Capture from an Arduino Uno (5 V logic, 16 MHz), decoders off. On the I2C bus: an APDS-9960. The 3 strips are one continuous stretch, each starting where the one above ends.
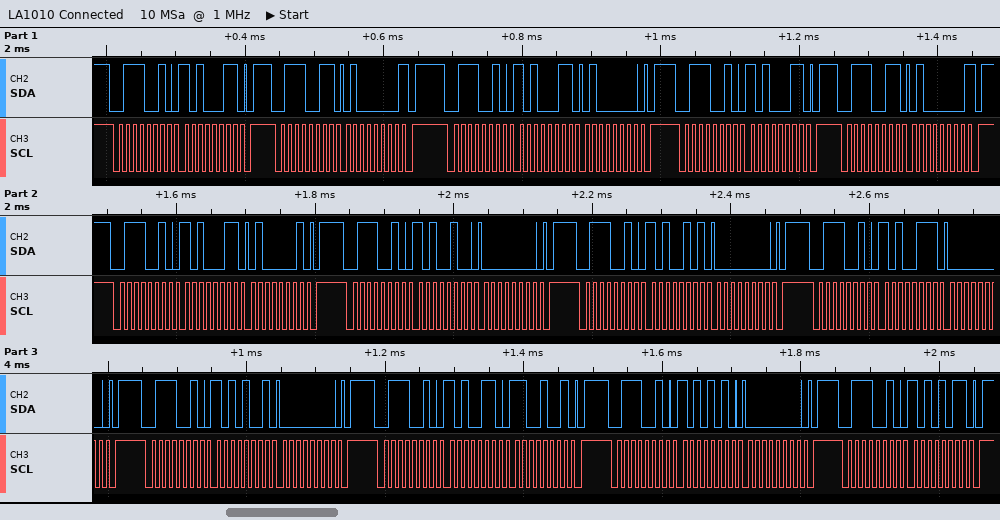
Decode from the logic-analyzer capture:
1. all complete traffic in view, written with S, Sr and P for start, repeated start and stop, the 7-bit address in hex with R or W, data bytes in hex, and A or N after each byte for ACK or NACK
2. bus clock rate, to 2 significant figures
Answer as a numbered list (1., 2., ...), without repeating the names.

1. S 39W A A3 A P S 39R A 40 N P S 39W A A3 A 40 A P S 39W A A3 A P S 39R A 40 N P S 39W A A3 A 41 A P S 39W A A4 A 00 A P S 39W A A5 A 00 A P S 39W A A7 A 00 A P S 39W A A9 A 00 A P S 39W A A6 A C9 A P S 39W A AA A 00 A P S 39W A AB A P
2. 100 kHz
